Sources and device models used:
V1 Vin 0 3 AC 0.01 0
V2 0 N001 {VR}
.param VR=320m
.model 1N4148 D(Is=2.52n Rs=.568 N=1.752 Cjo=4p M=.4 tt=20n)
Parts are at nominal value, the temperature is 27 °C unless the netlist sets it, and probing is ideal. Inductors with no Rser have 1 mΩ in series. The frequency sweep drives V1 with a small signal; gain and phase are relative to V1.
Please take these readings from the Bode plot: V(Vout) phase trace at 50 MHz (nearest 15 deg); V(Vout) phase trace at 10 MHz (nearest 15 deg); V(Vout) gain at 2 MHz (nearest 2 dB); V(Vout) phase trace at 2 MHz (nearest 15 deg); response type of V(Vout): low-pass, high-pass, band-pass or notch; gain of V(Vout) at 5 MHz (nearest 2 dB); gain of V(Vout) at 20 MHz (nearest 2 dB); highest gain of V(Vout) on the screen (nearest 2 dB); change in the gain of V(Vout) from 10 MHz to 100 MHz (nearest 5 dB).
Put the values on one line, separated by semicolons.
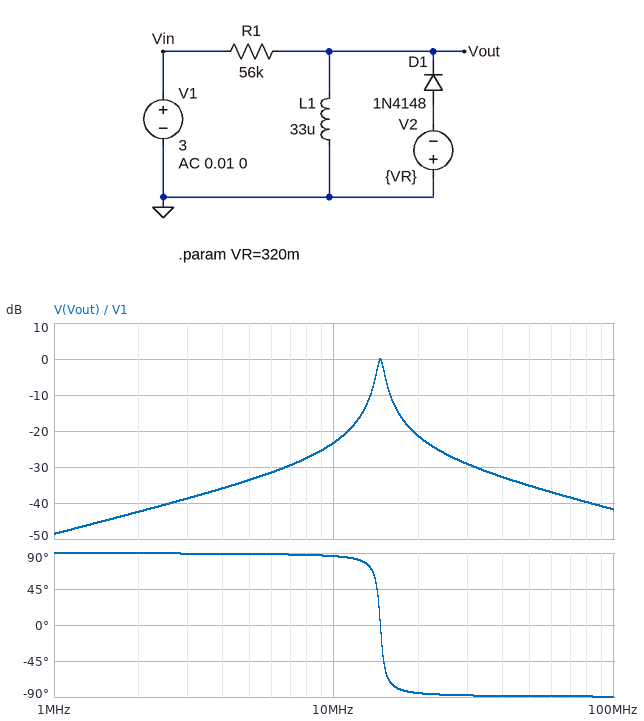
-90 deg; 90 deg; -42 dB; 90 deg; band-pass; -34 dB; -22 dB; 0 dB; -20 dB
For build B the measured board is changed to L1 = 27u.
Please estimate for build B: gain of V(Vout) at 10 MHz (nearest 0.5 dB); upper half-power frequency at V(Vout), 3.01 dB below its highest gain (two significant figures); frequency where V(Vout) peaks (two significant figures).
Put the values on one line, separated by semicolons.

-26.0 dB; 17 MHz; 16 MHz
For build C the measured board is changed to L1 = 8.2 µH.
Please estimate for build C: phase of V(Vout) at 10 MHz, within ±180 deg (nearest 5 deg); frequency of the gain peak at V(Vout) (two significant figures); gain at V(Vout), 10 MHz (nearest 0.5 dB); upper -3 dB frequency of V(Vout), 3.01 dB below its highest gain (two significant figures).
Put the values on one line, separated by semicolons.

90 deg; 29 MHz; -39.5 dB; 30 MHz
